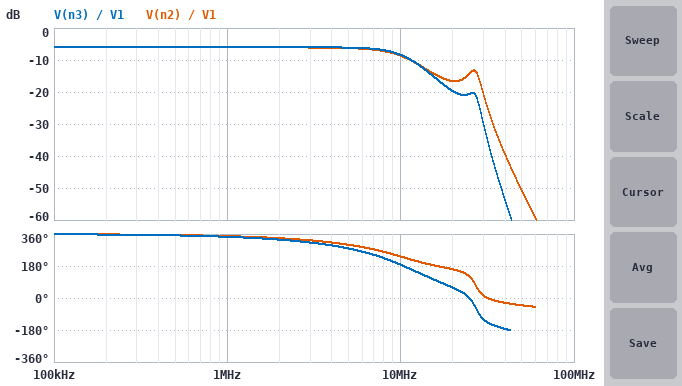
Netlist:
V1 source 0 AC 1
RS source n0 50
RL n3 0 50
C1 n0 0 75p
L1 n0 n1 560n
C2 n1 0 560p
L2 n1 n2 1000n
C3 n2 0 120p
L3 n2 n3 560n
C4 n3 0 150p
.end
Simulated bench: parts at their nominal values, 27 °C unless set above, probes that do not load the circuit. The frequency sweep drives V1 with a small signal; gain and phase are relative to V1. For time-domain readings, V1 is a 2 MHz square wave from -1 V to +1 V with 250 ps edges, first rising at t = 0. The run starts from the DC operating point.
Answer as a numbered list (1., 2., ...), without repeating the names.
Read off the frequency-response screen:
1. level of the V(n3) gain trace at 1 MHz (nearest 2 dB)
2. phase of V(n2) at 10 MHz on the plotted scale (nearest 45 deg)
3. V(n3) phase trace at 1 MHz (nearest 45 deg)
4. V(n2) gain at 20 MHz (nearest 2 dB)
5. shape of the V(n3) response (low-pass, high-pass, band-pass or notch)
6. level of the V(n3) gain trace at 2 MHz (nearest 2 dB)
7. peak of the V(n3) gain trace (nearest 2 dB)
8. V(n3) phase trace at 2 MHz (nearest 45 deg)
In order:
1. -6 dB
2. 225 deg
3. 360 deg
4. -16 dB
5. low-pass
6. -6 dB
7. -6 dB
8. 315 deg
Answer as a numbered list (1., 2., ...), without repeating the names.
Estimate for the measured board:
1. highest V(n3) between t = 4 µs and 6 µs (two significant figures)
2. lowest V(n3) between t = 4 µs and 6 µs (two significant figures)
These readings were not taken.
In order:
1. 580 mV
2. -580 mV
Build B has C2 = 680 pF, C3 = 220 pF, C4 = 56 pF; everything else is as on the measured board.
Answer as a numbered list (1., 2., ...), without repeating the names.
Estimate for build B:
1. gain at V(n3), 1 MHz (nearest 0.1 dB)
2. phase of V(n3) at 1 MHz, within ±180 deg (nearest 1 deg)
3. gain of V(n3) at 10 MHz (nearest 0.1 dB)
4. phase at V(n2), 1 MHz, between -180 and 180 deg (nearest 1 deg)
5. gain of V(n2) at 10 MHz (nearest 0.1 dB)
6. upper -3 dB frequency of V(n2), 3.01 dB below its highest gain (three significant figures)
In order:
1. -6.0 dB
2. -17 deg
3. -8.9 dB
4. -13 deg
5. -7.9 dB
6. 12.1 MHz
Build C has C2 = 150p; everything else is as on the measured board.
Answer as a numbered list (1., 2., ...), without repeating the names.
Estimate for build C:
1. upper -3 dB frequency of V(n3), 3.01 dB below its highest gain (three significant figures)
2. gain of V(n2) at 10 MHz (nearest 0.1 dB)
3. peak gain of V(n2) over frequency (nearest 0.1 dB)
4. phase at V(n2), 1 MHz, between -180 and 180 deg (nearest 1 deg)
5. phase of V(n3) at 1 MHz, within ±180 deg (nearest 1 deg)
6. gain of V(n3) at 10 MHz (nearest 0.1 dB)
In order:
1. 29.3 MHz
2. -7.6 dB
3. 1.3 dB
4. -8 deg
5. -12 deg
6. -7.3 dB
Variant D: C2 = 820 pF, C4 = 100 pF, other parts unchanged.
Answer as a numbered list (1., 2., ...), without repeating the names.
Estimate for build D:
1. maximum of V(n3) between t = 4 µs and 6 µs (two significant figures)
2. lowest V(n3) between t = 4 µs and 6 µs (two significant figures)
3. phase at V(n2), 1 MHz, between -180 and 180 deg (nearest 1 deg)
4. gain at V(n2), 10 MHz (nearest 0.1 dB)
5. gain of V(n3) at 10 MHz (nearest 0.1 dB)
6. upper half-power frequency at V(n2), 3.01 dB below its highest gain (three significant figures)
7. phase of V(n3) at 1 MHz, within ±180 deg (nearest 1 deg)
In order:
1. 540 mV
2. -540 mV
3. -14 deg
4. -11.0 dB
5. -11.4 dB
6. 8.27 MHz
7. -18 deg
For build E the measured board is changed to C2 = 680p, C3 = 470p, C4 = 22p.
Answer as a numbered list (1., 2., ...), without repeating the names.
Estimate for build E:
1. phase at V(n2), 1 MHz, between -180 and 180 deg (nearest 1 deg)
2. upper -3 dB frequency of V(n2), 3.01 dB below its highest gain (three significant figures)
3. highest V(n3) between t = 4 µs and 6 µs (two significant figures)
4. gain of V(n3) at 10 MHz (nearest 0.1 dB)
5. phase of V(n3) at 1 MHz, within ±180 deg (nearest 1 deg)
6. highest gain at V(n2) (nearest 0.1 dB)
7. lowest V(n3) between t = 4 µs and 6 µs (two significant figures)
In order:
1. -15 deg
2. 12.3 MHz
3. 610 mV
4. -6.7 dB
5. -19 deg
6. -5.2 dB
7. -610 mV
